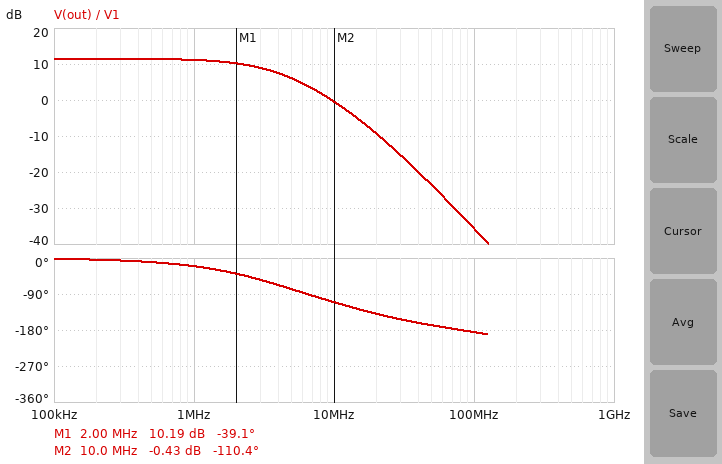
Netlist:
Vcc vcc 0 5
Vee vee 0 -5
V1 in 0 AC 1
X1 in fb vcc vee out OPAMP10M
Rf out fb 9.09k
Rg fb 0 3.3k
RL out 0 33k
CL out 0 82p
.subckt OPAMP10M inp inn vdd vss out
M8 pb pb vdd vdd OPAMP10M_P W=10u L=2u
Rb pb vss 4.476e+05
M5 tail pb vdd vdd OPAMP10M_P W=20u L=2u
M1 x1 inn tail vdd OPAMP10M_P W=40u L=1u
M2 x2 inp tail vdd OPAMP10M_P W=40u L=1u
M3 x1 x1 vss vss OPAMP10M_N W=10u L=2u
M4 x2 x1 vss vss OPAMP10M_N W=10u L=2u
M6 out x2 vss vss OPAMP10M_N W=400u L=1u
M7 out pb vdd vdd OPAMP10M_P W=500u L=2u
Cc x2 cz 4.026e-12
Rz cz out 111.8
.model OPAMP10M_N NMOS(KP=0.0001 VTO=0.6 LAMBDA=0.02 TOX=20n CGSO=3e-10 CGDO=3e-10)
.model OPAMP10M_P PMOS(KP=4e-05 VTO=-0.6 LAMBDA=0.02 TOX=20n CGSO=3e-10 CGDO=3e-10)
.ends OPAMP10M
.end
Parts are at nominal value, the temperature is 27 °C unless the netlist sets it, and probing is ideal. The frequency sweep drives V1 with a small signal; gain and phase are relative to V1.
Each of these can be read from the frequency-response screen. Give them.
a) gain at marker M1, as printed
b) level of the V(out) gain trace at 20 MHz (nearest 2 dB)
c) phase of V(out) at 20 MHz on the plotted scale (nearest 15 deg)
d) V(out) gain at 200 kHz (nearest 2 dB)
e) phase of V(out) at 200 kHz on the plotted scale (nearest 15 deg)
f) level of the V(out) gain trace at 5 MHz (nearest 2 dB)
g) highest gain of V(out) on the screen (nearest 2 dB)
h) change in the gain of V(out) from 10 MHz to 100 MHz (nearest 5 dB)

10.19 dB
-10 dB
-135 deg
12 dB
0 deg
6 dB
12 dB
-35 dB
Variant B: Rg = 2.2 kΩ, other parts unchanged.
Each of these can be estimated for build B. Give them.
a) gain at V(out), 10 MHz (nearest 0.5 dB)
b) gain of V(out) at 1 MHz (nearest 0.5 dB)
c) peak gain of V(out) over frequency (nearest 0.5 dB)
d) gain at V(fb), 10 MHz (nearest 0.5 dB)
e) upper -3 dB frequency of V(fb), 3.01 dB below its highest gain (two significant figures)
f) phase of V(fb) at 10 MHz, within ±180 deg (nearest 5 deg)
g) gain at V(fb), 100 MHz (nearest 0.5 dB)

-0.5 dB
13.5 dB
14.0 dB
-15.0 dB
2.3 MHz
-115 deg
-27.0 dB
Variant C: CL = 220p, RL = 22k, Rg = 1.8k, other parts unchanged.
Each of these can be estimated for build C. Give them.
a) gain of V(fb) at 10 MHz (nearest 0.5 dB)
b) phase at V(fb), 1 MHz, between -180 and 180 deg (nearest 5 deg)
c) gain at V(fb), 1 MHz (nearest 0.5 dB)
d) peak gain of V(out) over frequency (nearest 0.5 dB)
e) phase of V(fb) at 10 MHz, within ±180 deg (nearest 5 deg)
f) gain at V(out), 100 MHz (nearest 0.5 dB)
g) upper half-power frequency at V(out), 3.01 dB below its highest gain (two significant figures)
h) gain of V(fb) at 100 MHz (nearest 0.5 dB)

-20.5 dB
-35 deg
-0.5 dB
15.5 dB
-150 deg
-44.0 dB
2.2 MHz
-28.5 dB
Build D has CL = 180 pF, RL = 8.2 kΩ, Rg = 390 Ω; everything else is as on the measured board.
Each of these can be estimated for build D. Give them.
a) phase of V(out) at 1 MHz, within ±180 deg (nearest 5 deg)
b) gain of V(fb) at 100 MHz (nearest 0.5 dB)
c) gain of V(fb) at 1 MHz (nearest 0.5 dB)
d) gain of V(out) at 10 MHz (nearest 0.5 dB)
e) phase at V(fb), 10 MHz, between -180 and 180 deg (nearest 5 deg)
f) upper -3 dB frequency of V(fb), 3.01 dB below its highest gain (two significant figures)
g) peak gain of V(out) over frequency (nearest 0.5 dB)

-75 deg
-40.5 dB
-8.0 dB
-4.0 dB
-145 deg
440 kHz
27.5 dB
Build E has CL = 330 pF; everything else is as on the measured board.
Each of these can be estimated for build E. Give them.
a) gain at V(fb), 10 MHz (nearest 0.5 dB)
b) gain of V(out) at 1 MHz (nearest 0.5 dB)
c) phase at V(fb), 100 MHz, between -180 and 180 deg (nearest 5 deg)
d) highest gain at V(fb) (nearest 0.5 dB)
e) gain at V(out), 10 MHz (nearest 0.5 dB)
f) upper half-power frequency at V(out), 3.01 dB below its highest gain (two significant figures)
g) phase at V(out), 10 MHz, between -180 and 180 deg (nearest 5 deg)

-19.0 dB
11.5 dB
80 deg
0.5 dB
-7.5 dB
3.7 MHz
-155 deg
